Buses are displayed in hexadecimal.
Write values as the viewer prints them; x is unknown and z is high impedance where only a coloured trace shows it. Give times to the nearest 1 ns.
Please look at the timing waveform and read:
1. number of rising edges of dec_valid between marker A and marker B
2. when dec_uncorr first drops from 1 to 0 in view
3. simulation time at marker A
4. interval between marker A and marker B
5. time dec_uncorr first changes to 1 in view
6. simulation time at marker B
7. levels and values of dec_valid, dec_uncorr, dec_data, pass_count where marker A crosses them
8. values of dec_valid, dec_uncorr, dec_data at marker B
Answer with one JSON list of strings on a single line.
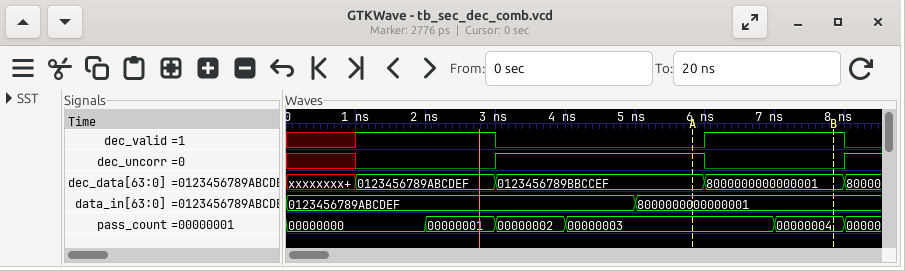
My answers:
["1", "6 ns", "6 ns", "2 ns", "3 ns", "8 ns", "dec_valid=0, dec_uncorr=1, dec_data=0123456789BBCCEF, pass_count=00000003", "dec_valid=1, dec_uncorr=0, dec_data=8000000000000001"]
